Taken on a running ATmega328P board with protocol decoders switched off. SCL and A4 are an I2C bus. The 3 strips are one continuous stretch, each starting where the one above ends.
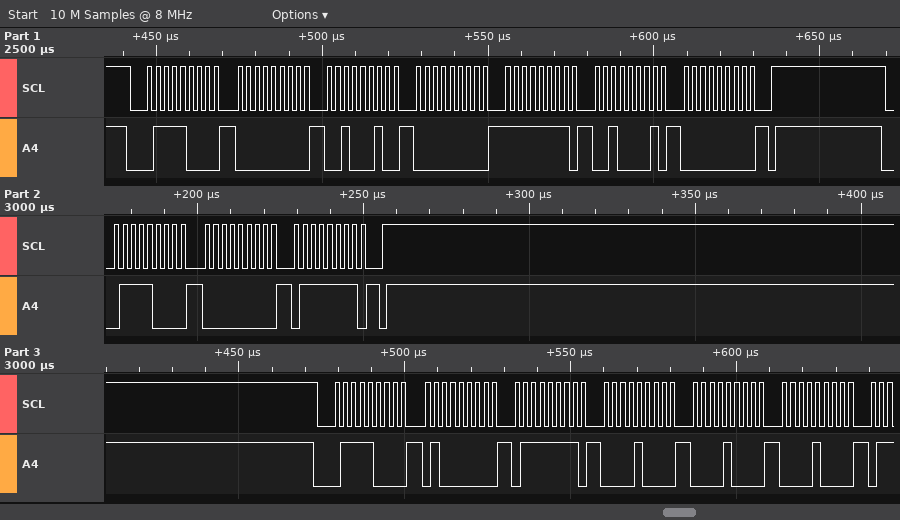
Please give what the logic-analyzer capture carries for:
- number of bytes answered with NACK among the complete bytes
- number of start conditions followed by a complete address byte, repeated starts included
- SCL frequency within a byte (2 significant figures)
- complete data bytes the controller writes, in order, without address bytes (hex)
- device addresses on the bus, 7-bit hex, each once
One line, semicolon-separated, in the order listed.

0; 3; 400 kHz; 00 22 00 FF 21 00 00 7F 40 7F 08 08 08; 0x3C
